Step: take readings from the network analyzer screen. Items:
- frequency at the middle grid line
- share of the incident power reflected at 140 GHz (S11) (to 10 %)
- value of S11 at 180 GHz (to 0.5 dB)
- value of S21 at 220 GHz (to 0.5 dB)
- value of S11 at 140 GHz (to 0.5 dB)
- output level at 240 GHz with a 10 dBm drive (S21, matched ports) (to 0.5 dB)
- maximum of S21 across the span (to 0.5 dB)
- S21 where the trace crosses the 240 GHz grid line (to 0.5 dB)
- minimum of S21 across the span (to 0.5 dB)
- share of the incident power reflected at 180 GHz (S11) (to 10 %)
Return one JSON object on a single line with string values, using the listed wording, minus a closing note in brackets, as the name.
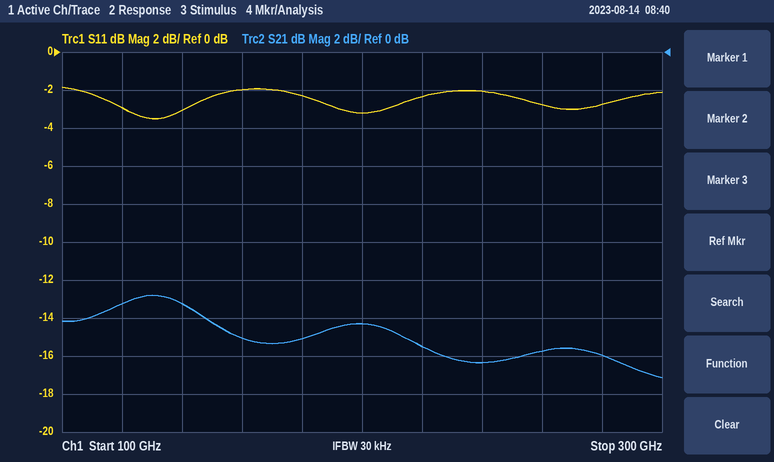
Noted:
{"frequency at the middle grid line": "200 GHz", "share of the incident power reflected at 140 GHz (S11)": "50 %", "value of S11 at 180 GHz": "-2.5 dB", "value of S21 at 220 GHz": "-15.5 dB", "value of S11 at 140 GHz": "-3.0 dB", "output level at 240 GHz with a 10 dBm drive (S21, matched ports)": "-6.5 dBm", "maximum of S21 across the span": "-13.0 dB", "S21 where the trace crosses the 240 GHz grid line": "-16.5 dB", "minimum of S21 across the span": "-17.0 dB", "share of the incident power reflected at 180 GHz (S11)": "60 %"}
